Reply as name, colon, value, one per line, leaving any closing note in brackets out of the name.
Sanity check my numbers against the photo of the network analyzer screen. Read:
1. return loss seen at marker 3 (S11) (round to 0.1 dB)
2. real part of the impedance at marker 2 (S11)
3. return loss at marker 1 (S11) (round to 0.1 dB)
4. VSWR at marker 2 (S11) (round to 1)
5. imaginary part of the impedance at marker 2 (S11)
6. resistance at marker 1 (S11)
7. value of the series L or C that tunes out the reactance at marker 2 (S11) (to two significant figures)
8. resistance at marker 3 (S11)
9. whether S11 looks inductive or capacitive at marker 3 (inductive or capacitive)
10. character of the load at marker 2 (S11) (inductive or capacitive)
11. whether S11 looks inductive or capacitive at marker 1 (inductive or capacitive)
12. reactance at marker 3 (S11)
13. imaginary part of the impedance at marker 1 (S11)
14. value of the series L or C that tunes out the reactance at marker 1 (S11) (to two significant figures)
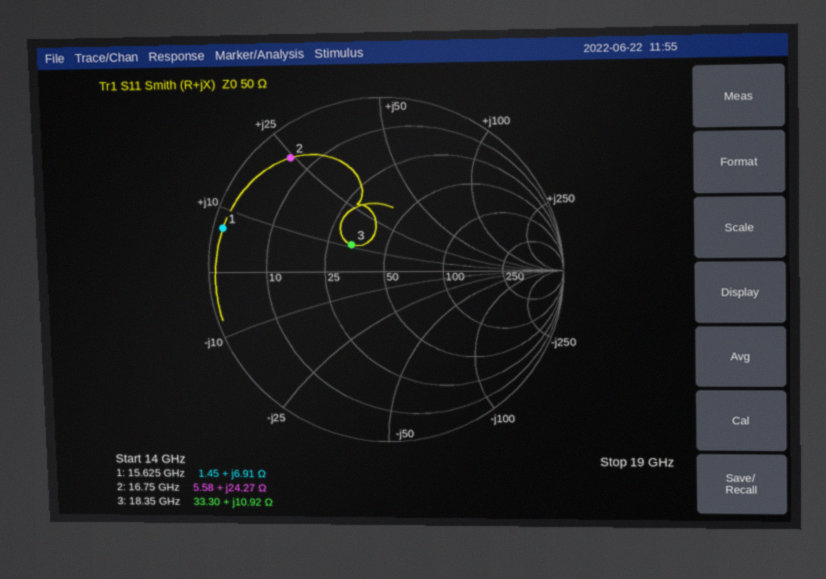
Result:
return loss seen at marker 3 (S11): 12.5 dB
real part of the impedance at marker 2: 5.58 Ω
return loss at marker 1 (S11): 0.5 dB
VSWR at marker 2 (S11): 11
imaginary part of the impedance at marker 2: +24.27 Ω
resistance at marker 1: 1.45 Ω
value of the series L or C that tunes out the reactance at marker 2 (S11): 390 fF
resistance at marker 3: 33.30 Ω
whether S11 looks inductive or capacitive at marker 3: inductive
character of the load at marker 2 (S11): inductive
whether S11 looks inductive or capacitive at marker 1: inductive
reactance at marker 3: +10.92 Ω
imaginary part of the impedance at marker 1: +6.91 Ω
value of the series L or C that tunes out the reactance at marker 1 (S11): 1.5 pF
